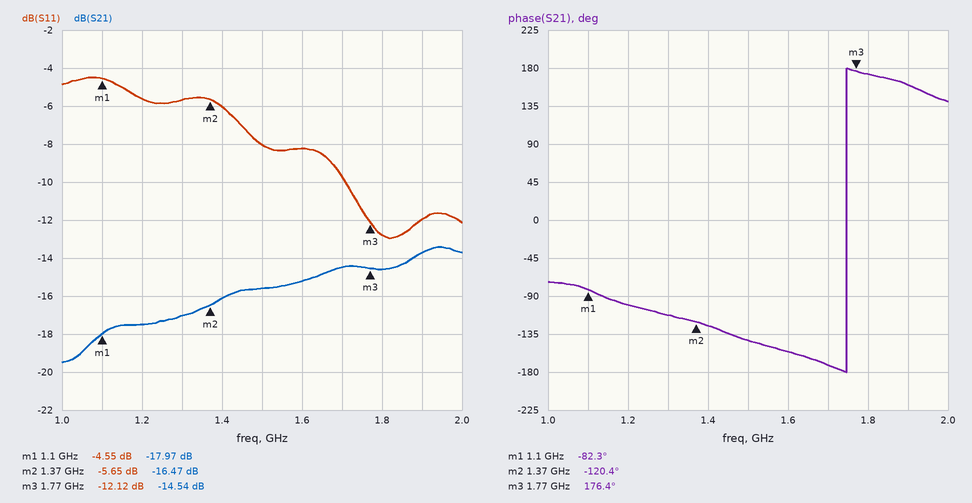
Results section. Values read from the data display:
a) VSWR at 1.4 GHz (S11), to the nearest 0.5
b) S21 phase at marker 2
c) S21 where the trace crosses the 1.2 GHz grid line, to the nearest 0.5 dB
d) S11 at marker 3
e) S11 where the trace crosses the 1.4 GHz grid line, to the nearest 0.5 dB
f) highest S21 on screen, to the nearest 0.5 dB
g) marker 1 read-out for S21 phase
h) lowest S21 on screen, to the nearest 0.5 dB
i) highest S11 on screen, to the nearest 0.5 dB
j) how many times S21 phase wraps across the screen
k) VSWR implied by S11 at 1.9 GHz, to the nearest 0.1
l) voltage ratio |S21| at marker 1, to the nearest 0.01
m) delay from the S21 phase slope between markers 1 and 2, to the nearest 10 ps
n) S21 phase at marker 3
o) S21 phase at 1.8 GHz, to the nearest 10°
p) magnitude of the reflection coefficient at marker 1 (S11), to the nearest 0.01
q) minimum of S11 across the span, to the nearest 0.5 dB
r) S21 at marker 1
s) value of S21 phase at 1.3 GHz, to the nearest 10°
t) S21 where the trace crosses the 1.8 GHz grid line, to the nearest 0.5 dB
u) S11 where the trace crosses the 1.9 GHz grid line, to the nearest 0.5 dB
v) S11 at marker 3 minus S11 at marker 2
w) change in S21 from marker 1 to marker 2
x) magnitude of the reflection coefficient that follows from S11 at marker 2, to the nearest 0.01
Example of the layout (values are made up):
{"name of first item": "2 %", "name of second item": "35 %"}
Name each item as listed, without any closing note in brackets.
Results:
{"VSWR at 1.4 GHz (S11), to the nearest 0.5": "3.0", "S21 phase at marker 2": "-120.4°", "S21 where the trace crosses the 1.2 GHz grid line, to the nearest 0.5 dB": "-17.5 dB", "S11 at marker 3": "-12.12 dB", "S11 where the trace crosses the 1.4 GHz grid line, to the nearest 0.5 dB": "-6.0 dB", "highest S21 on screen, to the nearest 0.5 dB": "-13.5 dB", "marker 1 read-out for S21 phase": "-82.3°", "lowest S21 on screen, to the nearest 0.5 dB": "-19.5 dB", "highest S11 on screen, to the nearest 0.5 dB": "-4.5 dB", "how many times S21 phase wraps across the screen": "1", "VSWR implied by S11 at 1.9 GHz, to the nearest 0.1": "1.7", "voltage ratio |S21| at marker 1, to the nearest 0.01": "0.13", "delay from the S21 phase slope between markers 1 and 2, to the nearest 10 ps": "390 ps", "S21 phase at marker 3": "176.4°", "S21 phase at 1.8 GHz, to the nearest 10°": "170°", "magnitude of the reflection coefficient at marker 1 (S11), to the nearest 0.01": "0.59", "minimum of S11 across the span, to the nearest 0.5 dB": "-13.0 dB", "S21 at marker 1": "-17.97 dB", "value of S21 phase at 1.3 GHz, to the nearest 10°": "-110°", "S21 where the trace crosses the 1.8 GHz grid line, to the nearest 0.5 dB": "-14.5 dB", "S11 where the trace crosses the 1.9 GHz grid line, to the nearest 0.5 dB": "-12.0 dB", "S11 at marker 3 minus S11 at marker 2": "-6.47 dB", "change in S21 from marker 1 to marker 2": "1.50 dB", "magnitude of the reflection coefficient that follows from S11 at marker 2, to the nearest 0.01": "0.52"}
